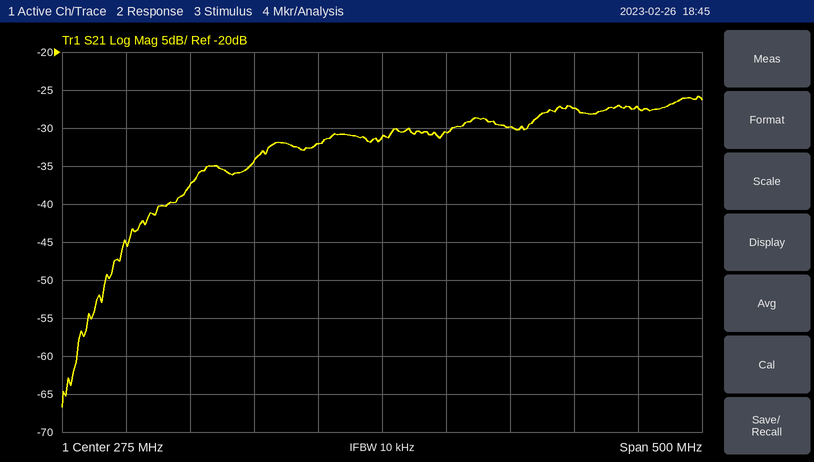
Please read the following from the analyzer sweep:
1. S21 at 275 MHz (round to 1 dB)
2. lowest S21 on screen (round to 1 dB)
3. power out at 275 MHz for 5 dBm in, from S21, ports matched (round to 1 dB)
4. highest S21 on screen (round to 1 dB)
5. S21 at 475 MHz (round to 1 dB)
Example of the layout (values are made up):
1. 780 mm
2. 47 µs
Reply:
1. -31 dB
2. -67 dB
3. -26 dBm
4. -26 dB
5. -27 dB
